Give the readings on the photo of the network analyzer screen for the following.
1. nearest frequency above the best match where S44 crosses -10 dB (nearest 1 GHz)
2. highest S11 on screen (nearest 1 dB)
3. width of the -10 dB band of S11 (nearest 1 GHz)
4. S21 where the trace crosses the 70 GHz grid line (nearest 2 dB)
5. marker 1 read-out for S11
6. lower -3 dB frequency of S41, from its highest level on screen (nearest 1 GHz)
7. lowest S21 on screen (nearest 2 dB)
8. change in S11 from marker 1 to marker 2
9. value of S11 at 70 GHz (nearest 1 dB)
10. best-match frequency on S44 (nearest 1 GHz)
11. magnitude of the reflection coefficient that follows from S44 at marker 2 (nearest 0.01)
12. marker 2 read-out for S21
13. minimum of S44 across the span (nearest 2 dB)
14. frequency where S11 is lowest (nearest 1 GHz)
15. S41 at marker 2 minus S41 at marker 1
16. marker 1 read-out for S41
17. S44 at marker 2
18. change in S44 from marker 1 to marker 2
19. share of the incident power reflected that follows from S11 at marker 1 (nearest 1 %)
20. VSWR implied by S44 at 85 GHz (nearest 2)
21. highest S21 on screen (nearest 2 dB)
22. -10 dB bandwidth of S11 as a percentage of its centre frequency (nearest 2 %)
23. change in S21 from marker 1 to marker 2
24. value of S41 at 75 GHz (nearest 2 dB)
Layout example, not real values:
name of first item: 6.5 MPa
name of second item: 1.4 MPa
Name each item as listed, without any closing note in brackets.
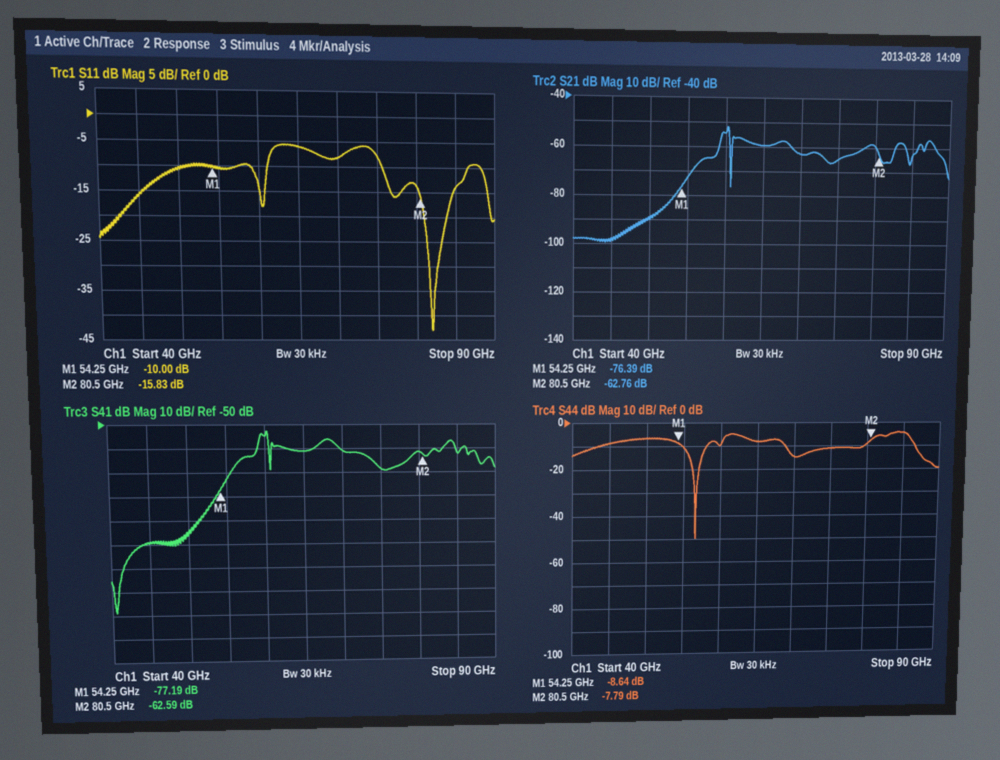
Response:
nearest frequency above the best match where S44 crosses -10 dB: 58 GHz
highest S11 on screen: -6 dB
width of the -10 dB band of S11: 11 GHz
S21 where the trace crosses the 70 GHz grid line: -62 dB
marker 1 read-out for S11: -10.00 dB
lower -3 dB frequency of S41, from its highest level on screen: 59 GHz
lowest S21 on screen: -100 dB
change in S11 from marker 1 to marker 2: -5.83 dB
value of S11 at 70 GHz: -8 dB
best-match frequency on S44: 57 GHz
magnitude of the reflection coefficient that follows from S44 at marker 2: 0.41
marker 2 read-out for S21: -62.76 dB
minimum of S44 across the span: -50 dB
frequency where S11 is lowest: 82 GHz
S41 at marker 2 minus S41 at marker 1: 14.60 dB
marker 1 read-out for S41: -77.19 dB
S44 at marker 2: -7.79 dB
change in S44 from marker 1 to marker 2: 0.85 dB
share of the incident power reflected that follows from S11 at marker 1: 10 %
VSWR implied by S44 at 85 GHz: 4
highest S21 on screen: -52 dB
-10 dB bandwidth of S11 as a percentage of its centre frequency: 14 %
change in S21 from marker 1 to marker 2: 13.63 dB
value of S41 at 75 GHz: -68 dB
